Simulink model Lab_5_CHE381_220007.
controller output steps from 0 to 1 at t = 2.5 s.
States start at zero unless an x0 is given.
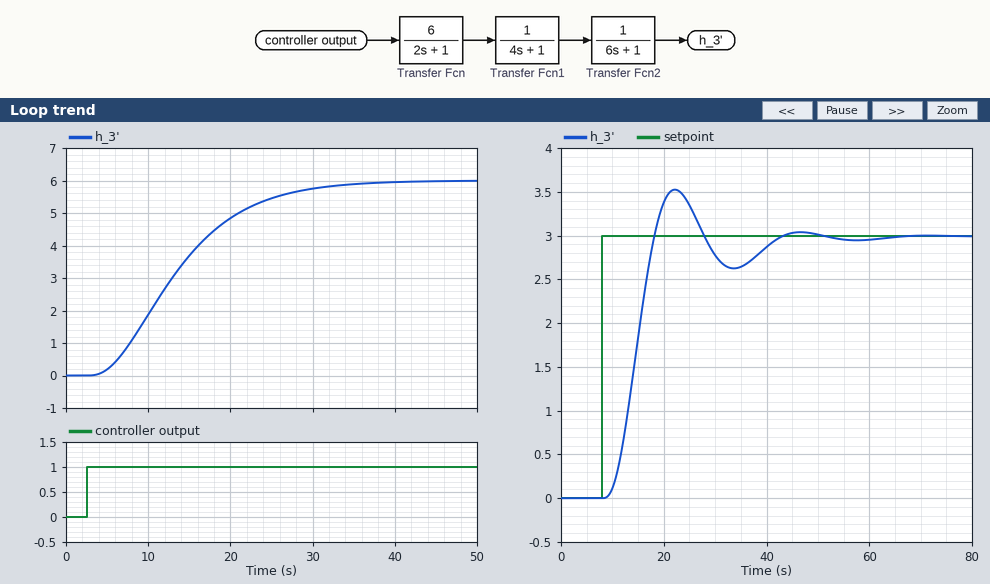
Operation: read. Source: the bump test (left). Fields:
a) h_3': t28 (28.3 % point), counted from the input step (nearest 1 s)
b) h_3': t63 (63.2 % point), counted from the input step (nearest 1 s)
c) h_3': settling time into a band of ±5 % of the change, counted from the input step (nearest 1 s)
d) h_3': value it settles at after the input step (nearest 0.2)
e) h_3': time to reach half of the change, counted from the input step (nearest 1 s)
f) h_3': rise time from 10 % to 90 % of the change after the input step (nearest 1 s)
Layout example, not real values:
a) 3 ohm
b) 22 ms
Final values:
a) 7 s
b) 13 s
c) 26 s
d) 6.0
e) 10 s
f) 18 s
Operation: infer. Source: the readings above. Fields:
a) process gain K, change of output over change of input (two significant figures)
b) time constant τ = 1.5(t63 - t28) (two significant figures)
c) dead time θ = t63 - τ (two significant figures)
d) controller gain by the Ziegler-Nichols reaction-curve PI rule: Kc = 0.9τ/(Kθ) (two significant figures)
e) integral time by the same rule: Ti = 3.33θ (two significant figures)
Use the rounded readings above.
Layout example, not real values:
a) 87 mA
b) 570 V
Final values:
a) 6.0
b) 9.0 s
c) 4.0 s
d) 0.34
e) 13 s
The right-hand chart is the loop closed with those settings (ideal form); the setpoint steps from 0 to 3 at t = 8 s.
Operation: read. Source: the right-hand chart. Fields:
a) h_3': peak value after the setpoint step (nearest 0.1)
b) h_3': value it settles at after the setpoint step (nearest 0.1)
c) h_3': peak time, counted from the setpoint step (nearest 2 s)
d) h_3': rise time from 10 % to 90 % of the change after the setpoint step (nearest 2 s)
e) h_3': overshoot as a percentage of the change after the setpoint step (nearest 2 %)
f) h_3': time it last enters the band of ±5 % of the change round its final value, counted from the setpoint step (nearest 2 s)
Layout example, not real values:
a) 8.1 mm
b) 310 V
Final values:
a) 3.5
b) 3.0
c) 14 s
d) 6 s
e) 18 %
f) 32 s
